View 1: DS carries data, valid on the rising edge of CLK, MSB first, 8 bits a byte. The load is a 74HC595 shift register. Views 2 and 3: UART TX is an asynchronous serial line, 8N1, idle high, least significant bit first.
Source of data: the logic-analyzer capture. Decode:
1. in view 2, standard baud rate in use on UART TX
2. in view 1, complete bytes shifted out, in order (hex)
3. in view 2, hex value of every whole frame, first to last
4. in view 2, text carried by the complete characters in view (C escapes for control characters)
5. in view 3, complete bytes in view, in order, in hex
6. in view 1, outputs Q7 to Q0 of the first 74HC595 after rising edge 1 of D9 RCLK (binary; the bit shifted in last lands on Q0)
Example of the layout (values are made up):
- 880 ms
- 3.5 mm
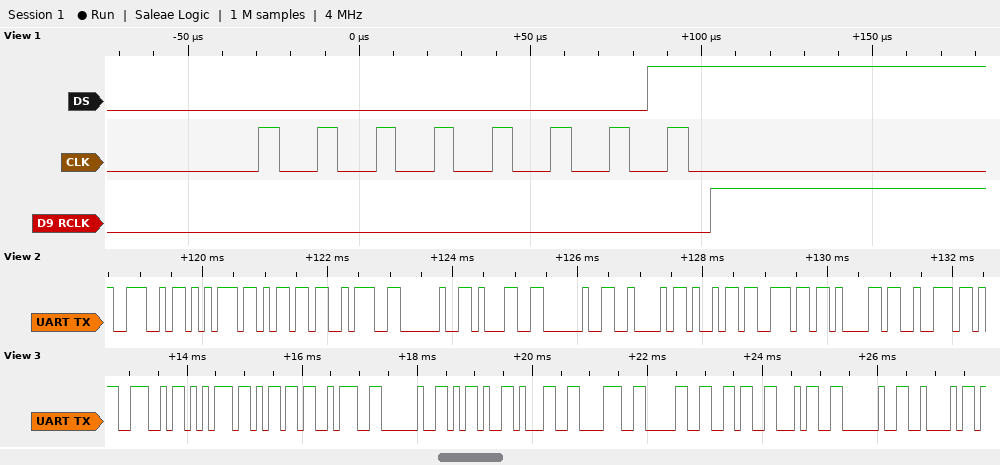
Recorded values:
- 9600 baud
- 0x01
- 4E 75 6D 3A 20 31 20 42 69 6E 61 72
- "Num: 1 Binar"
- 4E 75 6D 3A 20 2D 31 38 30 36 34 20 42
- 00000001
